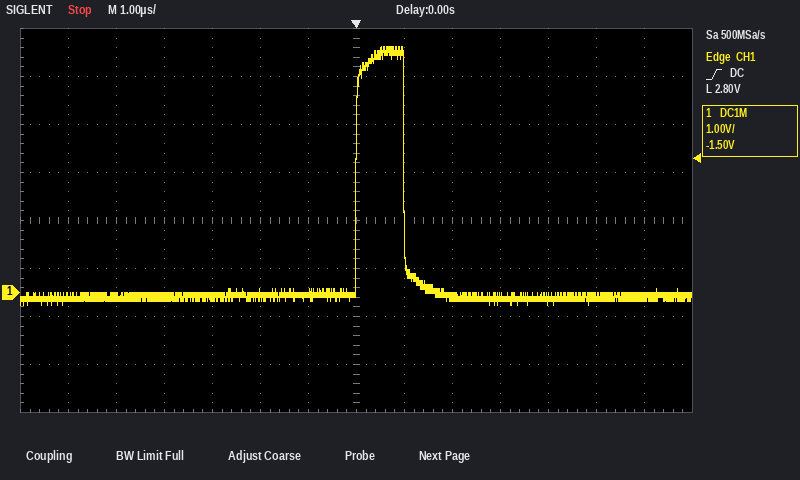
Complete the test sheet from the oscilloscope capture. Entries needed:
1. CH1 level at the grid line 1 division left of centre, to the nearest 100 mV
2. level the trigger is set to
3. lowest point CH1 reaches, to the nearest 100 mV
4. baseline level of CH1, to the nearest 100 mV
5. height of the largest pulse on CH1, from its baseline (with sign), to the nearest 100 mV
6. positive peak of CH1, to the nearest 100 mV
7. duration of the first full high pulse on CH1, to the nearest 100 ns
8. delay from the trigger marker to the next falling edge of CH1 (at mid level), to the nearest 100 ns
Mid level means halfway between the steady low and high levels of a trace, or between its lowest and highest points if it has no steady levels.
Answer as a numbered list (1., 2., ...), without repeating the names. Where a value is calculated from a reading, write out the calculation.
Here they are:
1. 0.0 V
2. 2.80 V
3. -200 mV
4. -100 mV
5. 5.1 V − (-100 mV) = +5.2 V
6. 5.1 V
7. 1.0 µs
8. 1.0 µs
